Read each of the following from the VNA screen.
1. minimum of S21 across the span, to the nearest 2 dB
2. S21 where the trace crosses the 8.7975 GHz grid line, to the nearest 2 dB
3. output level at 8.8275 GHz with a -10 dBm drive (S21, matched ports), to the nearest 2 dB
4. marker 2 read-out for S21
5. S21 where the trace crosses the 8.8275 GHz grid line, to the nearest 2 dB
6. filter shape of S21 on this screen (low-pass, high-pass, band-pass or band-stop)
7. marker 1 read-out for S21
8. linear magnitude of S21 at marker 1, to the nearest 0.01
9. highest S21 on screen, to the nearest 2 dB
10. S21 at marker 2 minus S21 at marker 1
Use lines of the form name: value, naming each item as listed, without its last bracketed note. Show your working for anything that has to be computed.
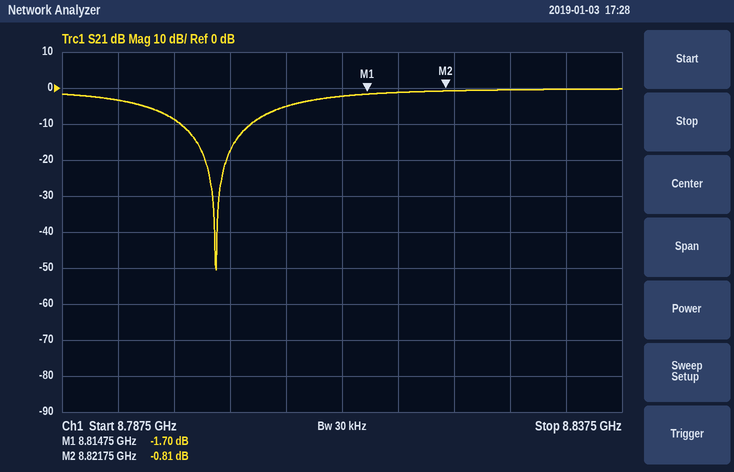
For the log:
minimum of S21 across the span, to the nearest 2 dB: -50 dB
S21 where the trace crosses the 8.7975 GHz grid line, to the nearest 2 dB: -8 dB
output level at 8.8275 GHz with a -10 dBm drive (S21, matched ports), to the nearest 2 dB: -10 dBm + (0 dB) = -10 dBm
marker 2 read-out for S21: -0.81 dB
S21 where the trace crosses the 8.8275 GHz grid line, to the nearest 2 dB: 0 dB
filter shape of S21 on this screen: band-stop
marker 1 read-out for S21: -1.70 dB
linear magnitude of S21 at marker 1, to the nearest 0.01: 10^(-1.7/20) ≈ 0.82
highest S21 on screen, to the nearest 2 dB: 0 dB
S21 at marker 2 minus S21 at marker 1: -0.81 − (-1.7) = 0.89 dB
